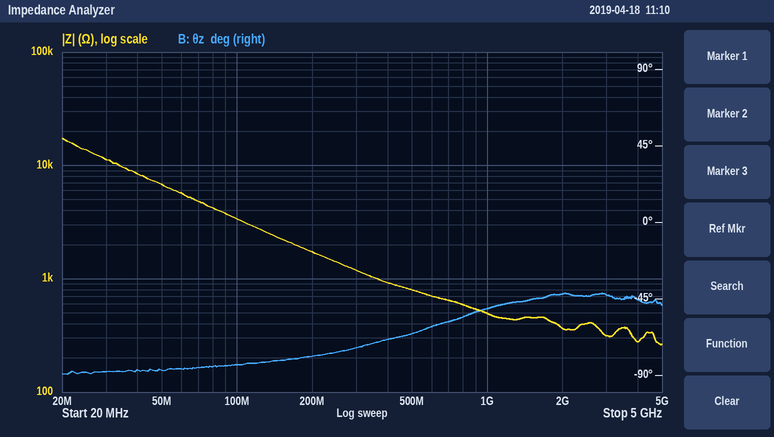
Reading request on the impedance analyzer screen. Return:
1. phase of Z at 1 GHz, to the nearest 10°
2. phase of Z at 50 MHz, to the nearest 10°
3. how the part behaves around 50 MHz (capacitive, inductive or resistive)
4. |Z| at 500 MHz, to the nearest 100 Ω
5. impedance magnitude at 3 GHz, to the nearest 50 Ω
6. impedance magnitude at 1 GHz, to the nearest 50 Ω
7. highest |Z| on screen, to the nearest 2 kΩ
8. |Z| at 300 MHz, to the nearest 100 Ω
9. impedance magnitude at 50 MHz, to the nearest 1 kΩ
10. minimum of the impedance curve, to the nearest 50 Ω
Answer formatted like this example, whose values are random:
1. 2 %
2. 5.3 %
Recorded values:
1. -50°
2. -90°
3. capacitive
4. 800 Ω
5. 300 Ω
6. 500 Ω
7. 18 kΩ
8. 1.2 kΩ
9. 7 kΩ
10. 250 Ω
